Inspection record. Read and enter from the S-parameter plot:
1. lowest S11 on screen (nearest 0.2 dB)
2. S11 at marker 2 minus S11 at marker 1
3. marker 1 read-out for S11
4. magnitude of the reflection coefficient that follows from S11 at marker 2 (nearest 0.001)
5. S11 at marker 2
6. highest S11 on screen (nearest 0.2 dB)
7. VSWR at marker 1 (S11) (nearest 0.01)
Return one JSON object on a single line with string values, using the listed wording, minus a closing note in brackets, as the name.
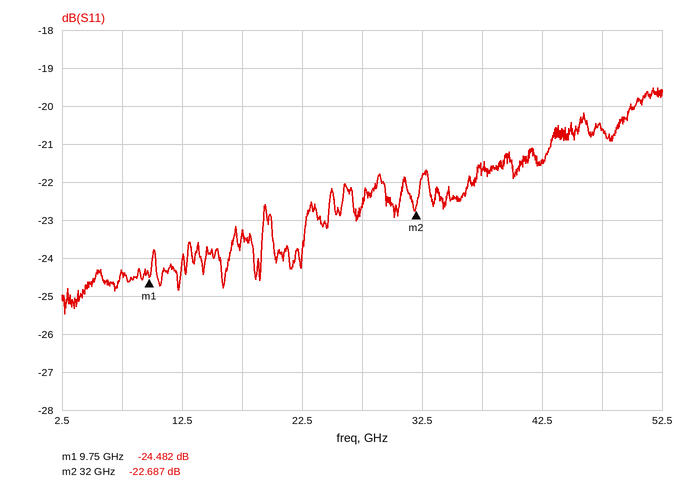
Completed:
{"lowest S11 on screen": "-25.4 dB", "S11 at marker 2 minus S11 at marker 1": "1.795 dB", "marker 1 read-out for S11": "-24.482 dB", "magnitude of the reflection coefficient that follows from S11 at marker 2": "0.073", "S11 at marker 2": "-22.687 dB", "highest S11 on screen": "-19.6 dB", "VSWR at marker 1 (S11)": "1.13"}
